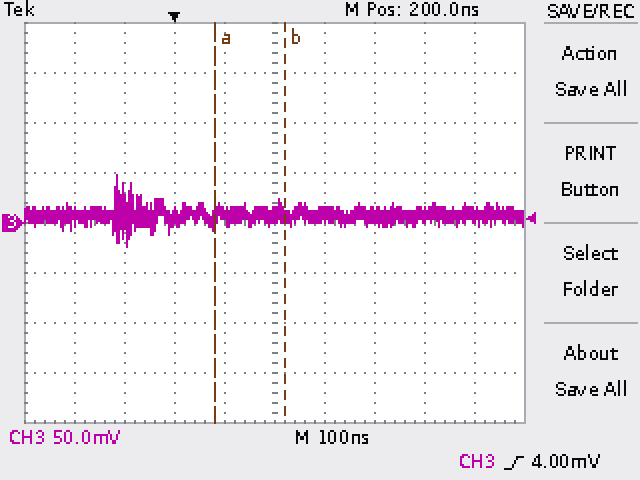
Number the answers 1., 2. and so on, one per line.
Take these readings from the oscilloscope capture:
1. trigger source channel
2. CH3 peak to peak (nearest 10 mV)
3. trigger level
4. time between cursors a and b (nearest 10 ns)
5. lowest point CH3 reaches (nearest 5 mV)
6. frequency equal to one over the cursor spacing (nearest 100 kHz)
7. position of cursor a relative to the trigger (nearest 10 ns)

1. CH3
2. 70 mV
3. 4.00 mV
4. 140 ns
5. -25 mV
6. 7.1 MHz
7. +80 ns
